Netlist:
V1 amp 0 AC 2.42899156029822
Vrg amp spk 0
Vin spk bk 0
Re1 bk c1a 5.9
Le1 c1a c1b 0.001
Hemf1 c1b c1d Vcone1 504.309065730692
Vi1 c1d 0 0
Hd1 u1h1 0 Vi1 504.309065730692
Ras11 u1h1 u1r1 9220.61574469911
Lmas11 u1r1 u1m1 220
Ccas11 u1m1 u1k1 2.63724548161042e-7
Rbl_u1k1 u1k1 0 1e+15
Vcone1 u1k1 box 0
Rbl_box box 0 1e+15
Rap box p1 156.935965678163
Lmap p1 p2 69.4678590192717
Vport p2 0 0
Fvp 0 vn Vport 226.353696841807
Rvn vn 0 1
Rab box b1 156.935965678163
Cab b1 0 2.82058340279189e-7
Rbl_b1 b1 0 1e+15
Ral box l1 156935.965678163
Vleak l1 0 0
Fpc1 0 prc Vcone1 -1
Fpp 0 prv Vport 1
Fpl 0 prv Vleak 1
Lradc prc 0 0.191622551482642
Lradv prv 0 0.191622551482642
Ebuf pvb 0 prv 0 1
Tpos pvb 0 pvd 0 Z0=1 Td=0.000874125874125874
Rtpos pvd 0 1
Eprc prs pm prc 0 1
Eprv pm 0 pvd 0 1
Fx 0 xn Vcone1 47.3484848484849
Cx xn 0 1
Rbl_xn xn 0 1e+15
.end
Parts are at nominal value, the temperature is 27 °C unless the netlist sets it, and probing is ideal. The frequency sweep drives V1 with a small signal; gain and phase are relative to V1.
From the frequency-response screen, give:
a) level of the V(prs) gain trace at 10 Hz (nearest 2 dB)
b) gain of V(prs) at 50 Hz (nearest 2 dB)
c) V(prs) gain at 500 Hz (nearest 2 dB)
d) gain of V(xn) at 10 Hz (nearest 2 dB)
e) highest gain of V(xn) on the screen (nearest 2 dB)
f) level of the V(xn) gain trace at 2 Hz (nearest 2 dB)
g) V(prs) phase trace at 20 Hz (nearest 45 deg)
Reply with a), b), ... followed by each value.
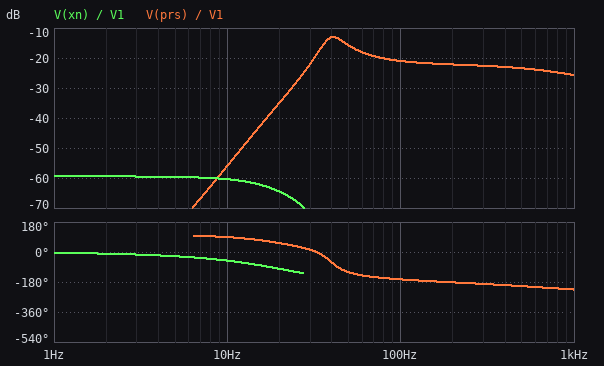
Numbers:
a) -56 dB
b) -16 dB
c) -24 dB
d) -60 dB
e) -60 dB
f) -60 dB
g) 45 deg
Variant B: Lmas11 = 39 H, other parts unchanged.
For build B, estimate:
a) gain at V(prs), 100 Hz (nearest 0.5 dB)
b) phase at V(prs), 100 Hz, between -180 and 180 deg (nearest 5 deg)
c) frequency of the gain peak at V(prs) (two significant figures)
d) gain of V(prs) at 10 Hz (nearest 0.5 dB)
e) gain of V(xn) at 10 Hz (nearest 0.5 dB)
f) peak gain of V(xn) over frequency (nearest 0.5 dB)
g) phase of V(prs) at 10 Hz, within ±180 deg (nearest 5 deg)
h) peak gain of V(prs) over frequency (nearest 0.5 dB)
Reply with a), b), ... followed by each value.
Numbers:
a) -13.0 dB
b) -105 deg
c) 420 Hz
d) -57.0 dB
e) -61.5 dB
f) -59.5 dB
g) 95 deg
h) -7.5 dB
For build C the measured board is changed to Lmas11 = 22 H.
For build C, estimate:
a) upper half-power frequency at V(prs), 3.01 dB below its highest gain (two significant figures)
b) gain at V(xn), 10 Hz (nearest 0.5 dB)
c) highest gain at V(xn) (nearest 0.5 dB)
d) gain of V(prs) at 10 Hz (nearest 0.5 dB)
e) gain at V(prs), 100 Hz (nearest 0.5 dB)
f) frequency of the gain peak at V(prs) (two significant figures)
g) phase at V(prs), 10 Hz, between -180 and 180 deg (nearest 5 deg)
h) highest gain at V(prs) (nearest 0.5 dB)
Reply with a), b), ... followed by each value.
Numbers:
a) 1.3 kHz
b) -61.5 dB
c) -59.5 dB
d) -57.0 dB
e) -13.0 dB
f) 580 Hz
g) 95 deg
h) -3.0 dB
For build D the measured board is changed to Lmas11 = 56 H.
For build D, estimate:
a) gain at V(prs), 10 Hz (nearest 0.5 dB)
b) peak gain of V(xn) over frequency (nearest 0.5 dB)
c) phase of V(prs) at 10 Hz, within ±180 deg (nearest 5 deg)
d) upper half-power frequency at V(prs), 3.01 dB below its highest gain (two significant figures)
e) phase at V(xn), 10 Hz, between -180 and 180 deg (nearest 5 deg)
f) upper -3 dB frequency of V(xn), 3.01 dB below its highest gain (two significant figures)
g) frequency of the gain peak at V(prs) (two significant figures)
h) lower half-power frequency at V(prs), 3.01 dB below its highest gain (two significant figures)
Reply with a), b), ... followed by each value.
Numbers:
a) -57.0 dB
b) -59.5 dB
c) 95 deg
d) 1.0 kHz
e) -45 deg
f) 14 Hz
g) 330 Hz
h) 95 Hz
